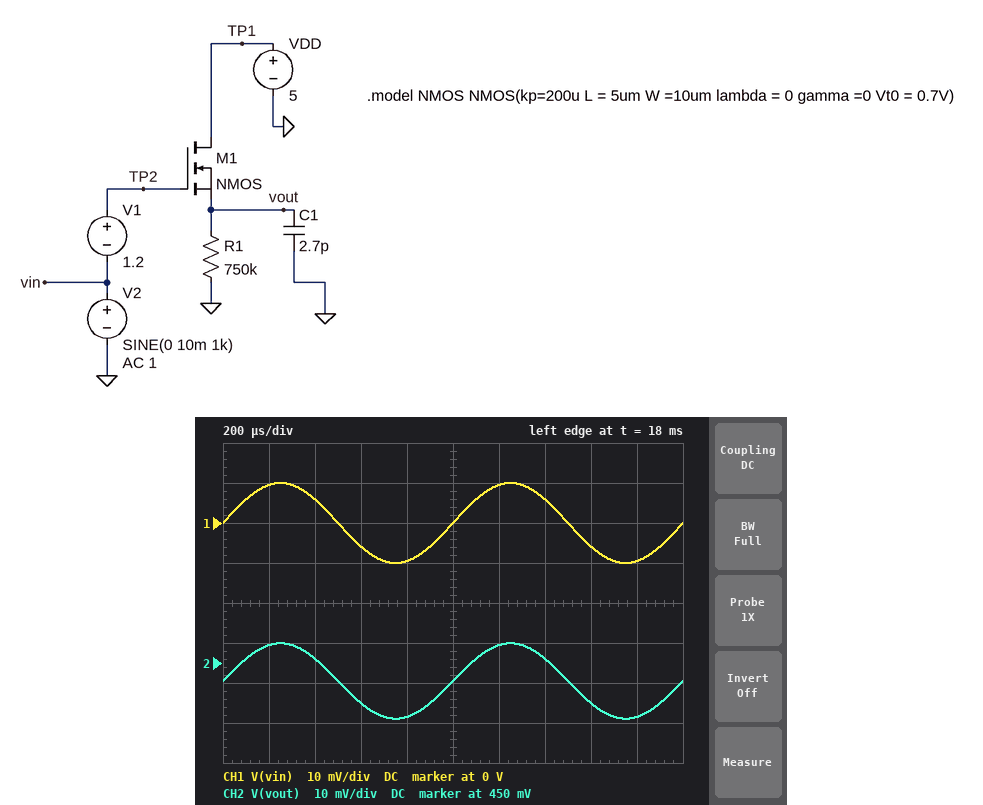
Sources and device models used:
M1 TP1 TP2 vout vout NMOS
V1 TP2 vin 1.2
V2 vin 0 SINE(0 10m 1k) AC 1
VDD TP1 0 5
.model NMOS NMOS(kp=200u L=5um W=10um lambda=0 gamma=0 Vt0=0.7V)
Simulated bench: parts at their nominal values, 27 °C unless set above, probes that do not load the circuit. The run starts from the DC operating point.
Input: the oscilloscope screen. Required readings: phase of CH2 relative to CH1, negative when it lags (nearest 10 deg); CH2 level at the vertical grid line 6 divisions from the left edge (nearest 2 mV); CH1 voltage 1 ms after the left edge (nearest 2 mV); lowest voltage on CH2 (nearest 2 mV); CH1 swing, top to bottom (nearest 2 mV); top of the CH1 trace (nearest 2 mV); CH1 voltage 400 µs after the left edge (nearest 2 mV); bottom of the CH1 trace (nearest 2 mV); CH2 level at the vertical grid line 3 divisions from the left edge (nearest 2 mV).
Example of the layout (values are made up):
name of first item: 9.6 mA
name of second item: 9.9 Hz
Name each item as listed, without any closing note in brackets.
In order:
phase of CH2 relative to CH1, negative when it lags: 0 deg
CH2 level at the vertical grid line 6 divisions from the left edge: 454 mV
CH1 voltage 1 ms after the left edge: 0 V
lowest voltage on CH2: 436 mV
CH1 swing, top to bottom: 20 mV
top of the CH1 trace: 10 mV
CH1 voltage 400 µs after the left edge: 6 mV
bottom of the CH1 trace: -10 mV
CH2 level at the vertical grid line 3 divisions from the left edge: 440 mV
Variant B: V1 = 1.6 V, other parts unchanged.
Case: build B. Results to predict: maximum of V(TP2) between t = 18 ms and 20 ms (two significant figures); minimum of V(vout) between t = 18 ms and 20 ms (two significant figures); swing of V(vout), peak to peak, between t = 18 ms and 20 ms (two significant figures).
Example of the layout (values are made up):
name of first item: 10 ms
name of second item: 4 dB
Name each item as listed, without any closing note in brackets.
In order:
maximum of V(TP2) between t = 18 ms and 20 ms: 1.6 V
minimum of V(vout) between t = 18 ms and 20 ms: 820 mV
swing of V(vout), peak to peak, between t = 18 ms and 20 ms: 19 mV
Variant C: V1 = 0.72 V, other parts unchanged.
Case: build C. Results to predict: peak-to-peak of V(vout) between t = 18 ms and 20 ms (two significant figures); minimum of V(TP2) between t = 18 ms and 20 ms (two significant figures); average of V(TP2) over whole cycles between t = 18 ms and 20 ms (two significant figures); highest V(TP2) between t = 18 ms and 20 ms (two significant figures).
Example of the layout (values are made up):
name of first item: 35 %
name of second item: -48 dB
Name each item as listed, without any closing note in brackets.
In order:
peak-to-peak of V(vout) between t = 18 ms and 20 ms: 14 mV
minimum of V(TP2) between t = 18 ms and 20 ms: 710 mV
average of V(TP2) over whole cycles between t = 18 ms and 20 ms: 720 mV
highest V(TP2) between t = 18 ms and 20 ms: 730 mV
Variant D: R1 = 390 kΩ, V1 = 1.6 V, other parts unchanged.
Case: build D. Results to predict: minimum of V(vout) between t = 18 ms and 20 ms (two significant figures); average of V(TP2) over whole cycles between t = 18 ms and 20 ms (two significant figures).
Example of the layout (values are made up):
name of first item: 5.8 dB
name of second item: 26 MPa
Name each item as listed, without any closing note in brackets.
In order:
minimum of V(vout) between t = 18 ms and 20 ms: 790 mV
average of V(TP2) over whole cycles between t = 18 ms and 20 ms: 1.6 V
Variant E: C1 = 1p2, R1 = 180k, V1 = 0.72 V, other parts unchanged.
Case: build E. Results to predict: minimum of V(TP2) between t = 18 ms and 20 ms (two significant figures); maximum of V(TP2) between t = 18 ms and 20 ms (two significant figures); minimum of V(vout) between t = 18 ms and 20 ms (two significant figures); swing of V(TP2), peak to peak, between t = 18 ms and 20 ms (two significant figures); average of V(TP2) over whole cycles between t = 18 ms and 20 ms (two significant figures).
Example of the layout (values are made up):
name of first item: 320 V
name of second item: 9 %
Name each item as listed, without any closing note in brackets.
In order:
minimum of V(TP2) between t = 18 ms and 20 ms: 710 mV
maximum of V(TP2) between t = 18 ms and 20 ms: 730 mV
minimum of V(vout) between t = 18 ms and 20 ms: 2.2 mV
swing of V(TP2), peak to peak, between t = 18 ms and 20 ms: 20 mV
average of V(TP2) over whole cycles between t = 18 ms and 20 ms: 720 mV
